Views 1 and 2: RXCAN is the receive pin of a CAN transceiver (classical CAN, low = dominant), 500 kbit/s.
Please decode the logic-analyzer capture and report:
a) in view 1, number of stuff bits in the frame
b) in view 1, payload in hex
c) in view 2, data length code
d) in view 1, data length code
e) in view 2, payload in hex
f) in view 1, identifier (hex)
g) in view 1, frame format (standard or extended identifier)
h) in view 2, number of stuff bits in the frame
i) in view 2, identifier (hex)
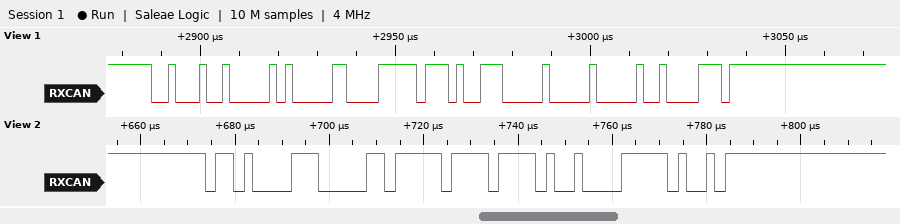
6
10 FF 4E 00
2
4
FF BD
0x224
standard
3
0x687
